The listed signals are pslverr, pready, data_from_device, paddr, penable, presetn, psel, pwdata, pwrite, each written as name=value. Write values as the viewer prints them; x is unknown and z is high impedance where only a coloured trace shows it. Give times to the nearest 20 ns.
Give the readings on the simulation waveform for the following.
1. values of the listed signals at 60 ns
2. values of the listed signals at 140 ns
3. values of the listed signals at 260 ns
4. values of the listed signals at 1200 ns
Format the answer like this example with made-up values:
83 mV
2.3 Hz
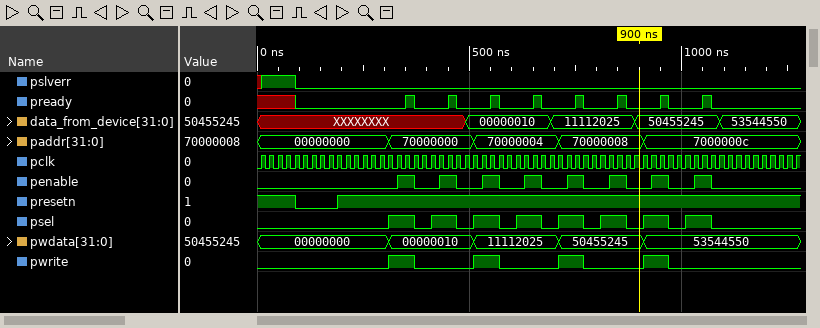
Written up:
pslverr=1, pready=x, data_from_device=XXXXXXXX, paddr=00000000, penable=0, presetn=1, psel=0, pwdata=00000000, pwrite=0
pslverr=0, pready=0, data_from_device=XXXXXXXX, paddr=00000000, penable=0, presetn=0, psel=0, pwdata=00000000, pwrite=0
pslverr=0, pready=0, data_from_device=XXXXXXXX, paddr=00000000, penable=0, presetn=1, psel=0, pwdata=00000000, pwrite=0
pslverr=0, pready=0, data_from_device=53544550, paddr=7000000c, penable=0, presetn=1, psel=0, pwdata=53544550, pwrite=0
